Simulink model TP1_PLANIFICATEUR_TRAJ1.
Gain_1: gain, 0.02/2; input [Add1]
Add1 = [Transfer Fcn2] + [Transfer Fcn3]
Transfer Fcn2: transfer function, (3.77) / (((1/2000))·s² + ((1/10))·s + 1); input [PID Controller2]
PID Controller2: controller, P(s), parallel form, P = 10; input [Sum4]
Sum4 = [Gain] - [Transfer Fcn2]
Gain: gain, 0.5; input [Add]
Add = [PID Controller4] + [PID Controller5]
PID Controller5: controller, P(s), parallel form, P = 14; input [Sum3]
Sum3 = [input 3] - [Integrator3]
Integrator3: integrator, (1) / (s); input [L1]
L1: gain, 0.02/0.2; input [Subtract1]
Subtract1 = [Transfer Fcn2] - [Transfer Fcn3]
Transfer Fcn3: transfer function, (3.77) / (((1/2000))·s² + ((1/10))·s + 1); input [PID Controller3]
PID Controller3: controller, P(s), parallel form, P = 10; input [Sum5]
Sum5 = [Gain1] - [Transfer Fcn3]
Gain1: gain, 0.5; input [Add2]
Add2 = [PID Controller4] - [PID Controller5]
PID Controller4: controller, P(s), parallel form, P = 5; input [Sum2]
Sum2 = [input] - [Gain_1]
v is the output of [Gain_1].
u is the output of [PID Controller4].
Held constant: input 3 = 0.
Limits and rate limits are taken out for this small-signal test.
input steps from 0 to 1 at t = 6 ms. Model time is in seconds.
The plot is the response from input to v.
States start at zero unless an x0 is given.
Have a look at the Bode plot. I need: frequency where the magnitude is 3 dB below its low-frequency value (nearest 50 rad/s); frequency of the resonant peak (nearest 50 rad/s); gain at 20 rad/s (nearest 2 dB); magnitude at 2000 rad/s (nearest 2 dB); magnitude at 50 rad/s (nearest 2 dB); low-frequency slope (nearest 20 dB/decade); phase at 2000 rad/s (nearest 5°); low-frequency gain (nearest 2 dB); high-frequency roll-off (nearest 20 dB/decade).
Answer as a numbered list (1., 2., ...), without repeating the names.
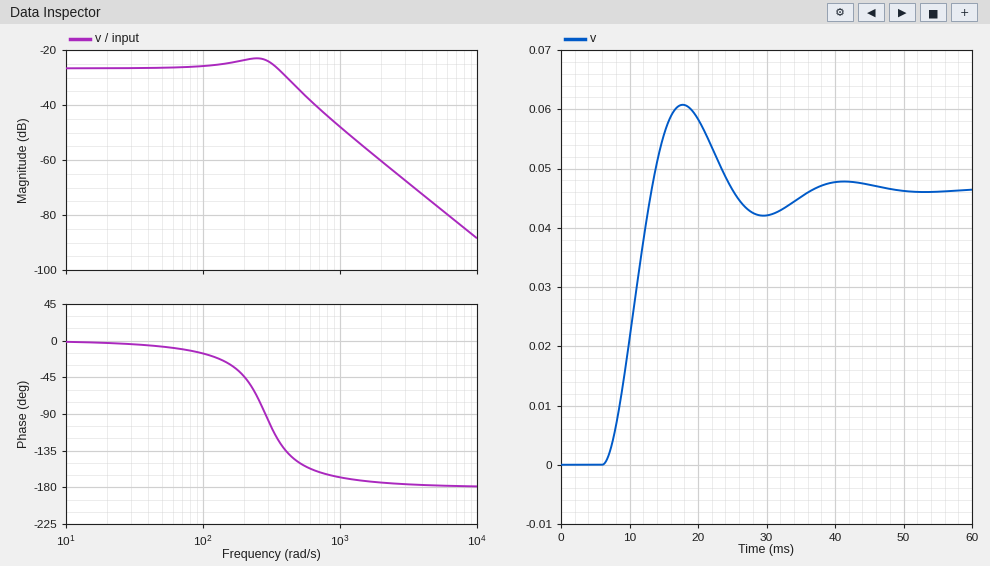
1. 400 rad/s
2. 250 rad/s
3. -26 dB
4. -60 dB
5. -26 dB
6. 0 dB/decade
7. -175°
8. -26 dB
9. -40 dB/decade
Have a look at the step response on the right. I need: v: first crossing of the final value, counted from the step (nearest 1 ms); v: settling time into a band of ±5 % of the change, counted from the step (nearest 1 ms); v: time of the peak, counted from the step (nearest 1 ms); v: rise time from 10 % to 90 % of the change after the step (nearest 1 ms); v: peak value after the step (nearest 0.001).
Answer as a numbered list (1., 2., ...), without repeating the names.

1. 7 ms
2. 28 ms
3. 12 ms
4. 5 ms
5. 0.061
